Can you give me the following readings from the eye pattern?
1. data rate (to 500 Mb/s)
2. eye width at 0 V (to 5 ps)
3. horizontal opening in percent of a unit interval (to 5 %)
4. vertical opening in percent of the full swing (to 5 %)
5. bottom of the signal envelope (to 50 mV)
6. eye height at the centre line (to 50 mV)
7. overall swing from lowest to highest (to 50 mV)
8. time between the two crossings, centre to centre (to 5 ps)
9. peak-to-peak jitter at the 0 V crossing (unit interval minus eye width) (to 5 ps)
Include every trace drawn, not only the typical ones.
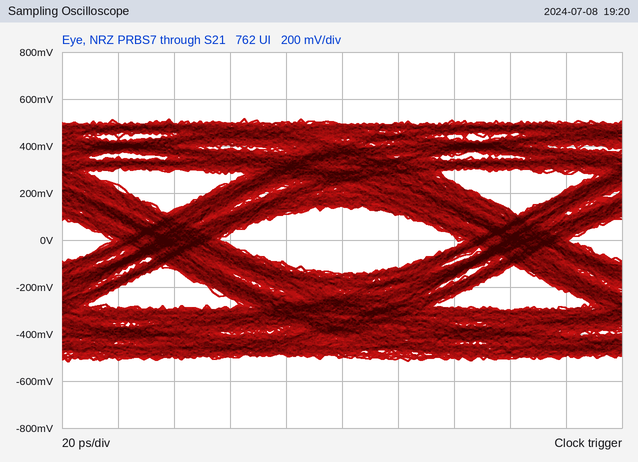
8.0 Gb/s
85 ps
70 %
30 %
-500 mV
300 mV
1.05 V
125 ps
40 ps
